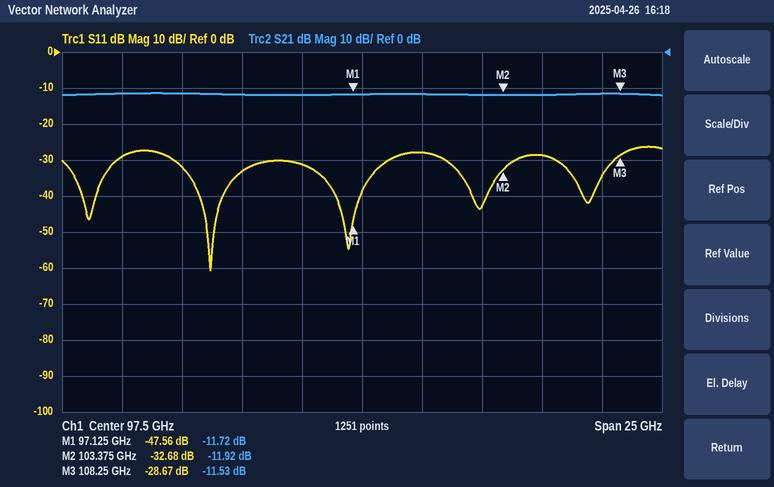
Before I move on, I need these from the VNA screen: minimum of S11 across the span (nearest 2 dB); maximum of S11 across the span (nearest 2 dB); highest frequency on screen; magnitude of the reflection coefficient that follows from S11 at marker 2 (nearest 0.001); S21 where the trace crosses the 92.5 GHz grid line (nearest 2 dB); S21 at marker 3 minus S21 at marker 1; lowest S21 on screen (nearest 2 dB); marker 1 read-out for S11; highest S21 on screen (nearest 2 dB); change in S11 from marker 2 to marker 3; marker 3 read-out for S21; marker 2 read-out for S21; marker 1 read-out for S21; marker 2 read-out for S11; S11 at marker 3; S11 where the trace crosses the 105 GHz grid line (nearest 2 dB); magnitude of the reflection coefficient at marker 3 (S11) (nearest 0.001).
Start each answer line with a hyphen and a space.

- -60 dB
- -26 dB
- 110 GHz
- 0.023
- -12 dB
- 0.19 dB
- -12 dB
- -47.56 dB
- -12 dB
- 4.01 dB
- -11.53 dB
- -11.92 dB
- -11.72 dB
- -32.68 dB
- -28.67 dB
- -28 dB
- 0.037
